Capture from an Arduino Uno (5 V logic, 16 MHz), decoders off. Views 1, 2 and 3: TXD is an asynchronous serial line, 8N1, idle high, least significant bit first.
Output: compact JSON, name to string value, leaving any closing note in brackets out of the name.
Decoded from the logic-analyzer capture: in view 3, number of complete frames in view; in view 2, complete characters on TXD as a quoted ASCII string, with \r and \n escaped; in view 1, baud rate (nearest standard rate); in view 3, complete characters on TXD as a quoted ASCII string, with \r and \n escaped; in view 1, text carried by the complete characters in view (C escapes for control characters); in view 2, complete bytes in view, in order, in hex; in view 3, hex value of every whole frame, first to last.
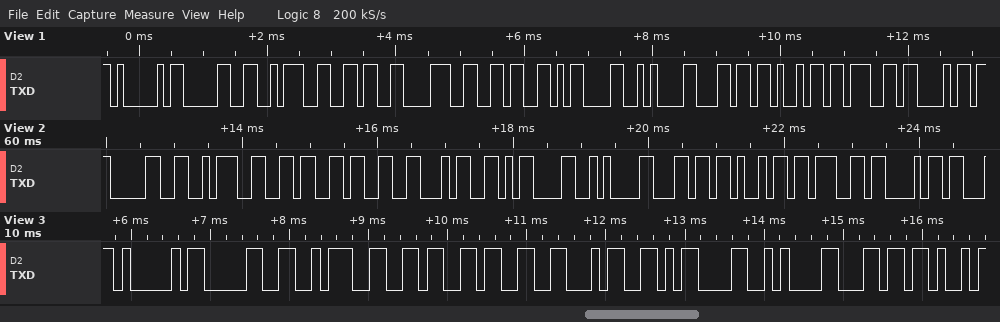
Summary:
{"in view 3, number of complete frames in view": "9", "in view 2, complete characters on TXD as a quoted ASCII string, with \\r and \\n escaped": "\"0:634\\r\\nligh\"", "in view 1, baud rate": "9600 baud", "in view 3, complete characters on TXD as a quoted ASCII string, with \\r and \\n escaped": "\"A0:634\\r\\nl\"", "in view 1, text carried by the complete characters in view": "\"A0:686\\r\\nligh\"", "in view 2, complete bytes in view, in order, in hex": "30 3A 36 33 34 0D 0A 6C 69 67 68", "in view 3, hex value of every whole frame, first to last": "0x41 0x30 0x3A 0x36 0x33 0x34 0x0D 0x0A 0x6C"}
